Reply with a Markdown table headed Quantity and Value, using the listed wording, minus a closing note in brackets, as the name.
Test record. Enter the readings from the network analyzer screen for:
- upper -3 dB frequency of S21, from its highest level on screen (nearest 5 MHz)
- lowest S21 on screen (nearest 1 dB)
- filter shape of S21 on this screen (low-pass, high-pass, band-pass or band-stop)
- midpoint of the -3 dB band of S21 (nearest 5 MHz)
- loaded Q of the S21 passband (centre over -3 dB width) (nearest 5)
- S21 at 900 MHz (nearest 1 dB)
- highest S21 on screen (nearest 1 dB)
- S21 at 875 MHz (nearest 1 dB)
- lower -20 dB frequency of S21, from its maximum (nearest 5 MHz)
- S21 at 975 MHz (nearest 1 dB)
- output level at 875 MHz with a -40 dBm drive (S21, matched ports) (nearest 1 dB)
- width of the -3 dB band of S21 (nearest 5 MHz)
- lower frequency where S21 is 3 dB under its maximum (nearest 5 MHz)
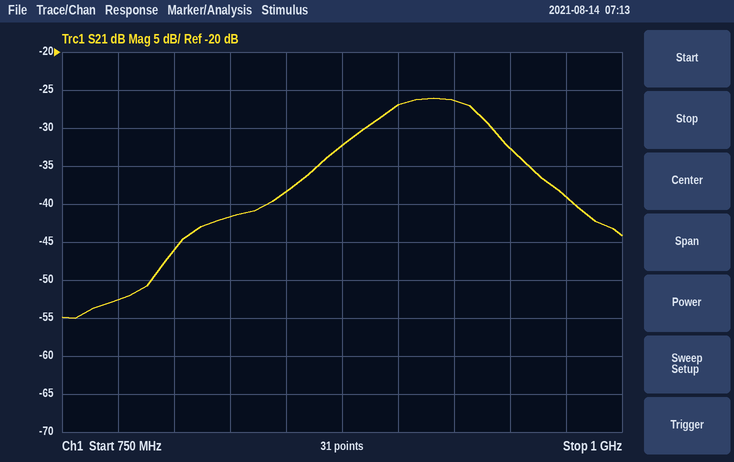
| Quantity | Value |
|---|---|
| upper -3 dB frequency of S21, from its highest level on screen | 940 MHz |
| lowest S21 on screen | -55 dB |
| filter shape of S21 on this screen | band-pass |
| midpoint of the -3 dB band of S21 | 915 MHz |
| loaded Q of the S21 passband (centre over -3 dB width) | 20 |
| S21 at 900 MHz | -27 dB |
| highest S21 on screen | -26 dB |
| S21 at 875 MHz | -32 dB |
| lower -20 dB frequency of S21, from its maximum | 800 MHz |
| S21 at 975 MHz | -39 dB |
| output level at 875 MHz with a -40 dBm drive (S21, matched ports) | -72 dBm |
| width of the -3 dB band of S21 | 50 MHz |
| lower frequency where S21 is 3 dB under its maximum | 890 MHz |
